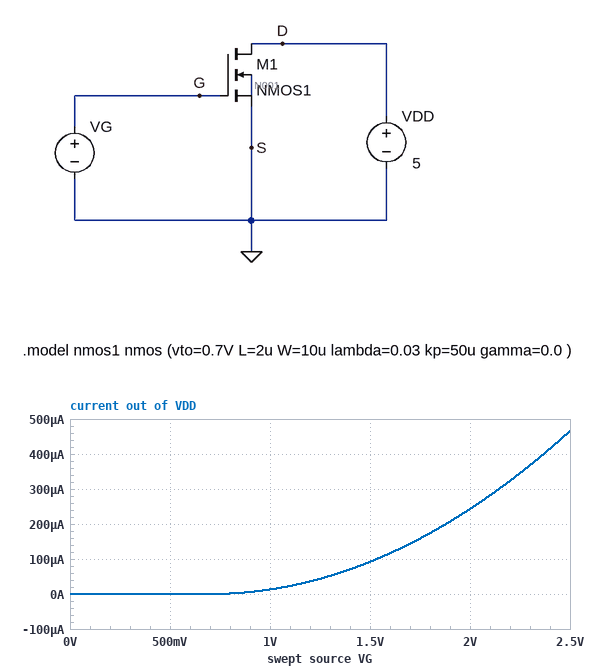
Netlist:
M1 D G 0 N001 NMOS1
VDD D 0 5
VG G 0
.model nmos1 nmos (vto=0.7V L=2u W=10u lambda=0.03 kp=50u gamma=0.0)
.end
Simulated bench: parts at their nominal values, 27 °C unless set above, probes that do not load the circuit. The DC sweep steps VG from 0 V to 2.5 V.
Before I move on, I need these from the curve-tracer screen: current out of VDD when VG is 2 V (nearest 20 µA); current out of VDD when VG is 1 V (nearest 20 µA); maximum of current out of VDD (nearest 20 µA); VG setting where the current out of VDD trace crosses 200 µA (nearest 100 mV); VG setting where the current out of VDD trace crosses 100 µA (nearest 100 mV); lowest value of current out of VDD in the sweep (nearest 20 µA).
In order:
240 µA
20 µA
460 µA
1.9 V
1.5 V
0 A
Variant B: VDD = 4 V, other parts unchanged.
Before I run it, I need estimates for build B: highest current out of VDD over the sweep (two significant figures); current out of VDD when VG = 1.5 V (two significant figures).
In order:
450 µA
90 µA
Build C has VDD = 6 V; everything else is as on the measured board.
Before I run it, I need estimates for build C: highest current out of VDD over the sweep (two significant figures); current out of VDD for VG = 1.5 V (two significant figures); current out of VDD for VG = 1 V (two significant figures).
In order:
480 µA
94 µA
13 µA
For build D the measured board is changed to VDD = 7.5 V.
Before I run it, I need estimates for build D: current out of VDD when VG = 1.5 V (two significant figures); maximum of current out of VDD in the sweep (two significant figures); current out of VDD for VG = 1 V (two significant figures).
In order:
98 µA
500 µA
14 µA
